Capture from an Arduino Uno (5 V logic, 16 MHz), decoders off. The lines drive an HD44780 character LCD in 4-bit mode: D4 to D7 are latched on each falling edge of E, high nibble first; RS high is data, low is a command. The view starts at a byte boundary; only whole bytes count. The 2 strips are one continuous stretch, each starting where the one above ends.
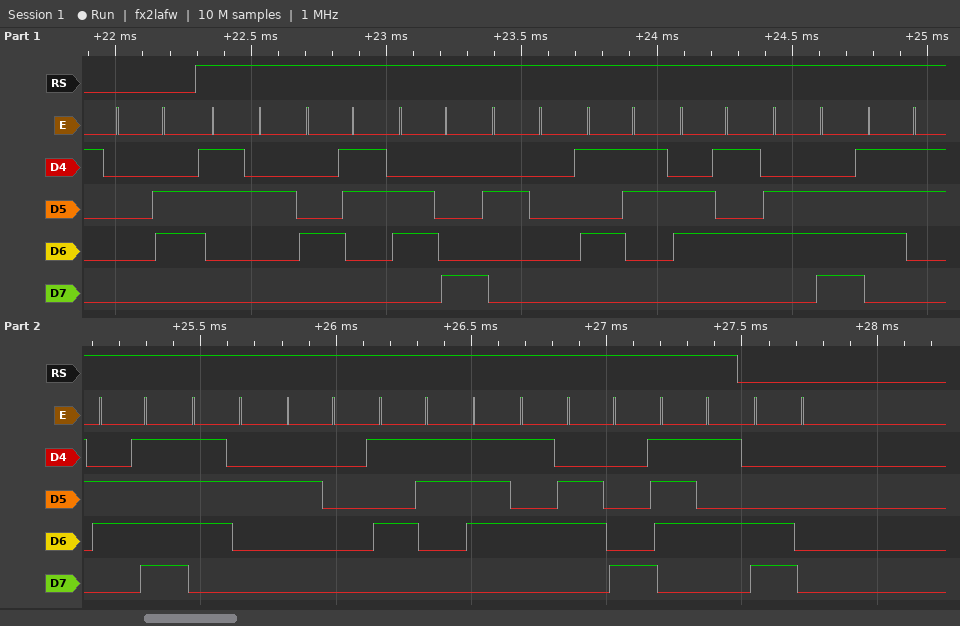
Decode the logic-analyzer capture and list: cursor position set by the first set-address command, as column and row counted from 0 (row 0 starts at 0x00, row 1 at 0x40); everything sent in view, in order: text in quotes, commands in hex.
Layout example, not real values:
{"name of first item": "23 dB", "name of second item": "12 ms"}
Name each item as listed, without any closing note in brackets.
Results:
{"cursor position set by the first set-address command, as column and row counted from 0": "column 0, row 1", "everything sent in view, in order: text in quotes, commands in hex": "0x06 \"2Ch Sensor Suhu\" 0xC0"}
